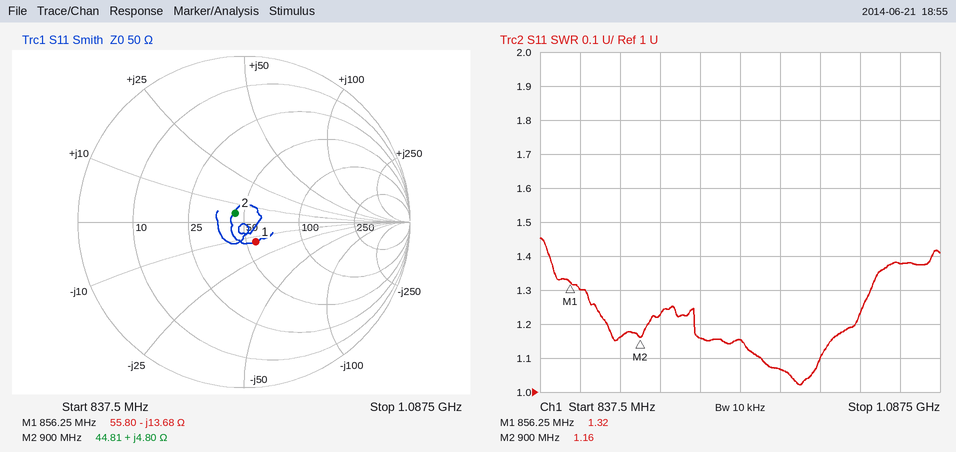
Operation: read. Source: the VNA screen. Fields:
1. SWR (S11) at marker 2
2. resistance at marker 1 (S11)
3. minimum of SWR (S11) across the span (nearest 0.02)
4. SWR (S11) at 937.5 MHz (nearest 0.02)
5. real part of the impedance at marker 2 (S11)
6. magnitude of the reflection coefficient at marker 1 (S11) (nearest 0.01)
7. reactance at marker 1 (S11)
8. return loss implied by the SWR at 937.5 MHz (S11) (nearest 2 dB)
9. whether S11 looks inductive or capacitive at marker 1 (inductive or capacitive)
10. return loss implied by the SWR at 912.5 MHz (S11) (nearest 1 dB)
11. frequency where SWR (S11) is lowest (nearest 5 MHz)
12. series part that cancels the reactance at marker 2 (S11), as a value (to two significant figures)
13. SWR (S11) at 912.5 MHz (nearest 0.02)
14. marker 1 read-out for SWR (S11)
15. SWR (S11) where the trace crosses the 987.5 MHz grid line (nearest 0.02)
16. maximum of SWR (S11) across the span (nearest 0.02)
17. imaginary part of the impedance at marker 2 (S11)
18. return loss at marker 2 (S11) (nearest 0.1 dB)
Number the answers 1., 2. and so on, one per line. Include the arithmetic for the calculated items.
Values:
1. 1.16
2. 55.80 Ω
3. 1.02
4. 1.16
5. 44.81 Ω
6. 0.14
7. -13.68 Ω
8. −20 log10((1.16 − 1)/(1.16 + 1)) ≈ 22.6 dB, so 22 dB to the nearest 2 dB
9. capacitive
10. −20 log10((1.22 − 1)/(1.22 + 1)) ≈ 20 dB
11. 1.000 GHz
12. C = 1/(2π × 900 MHz × 4.8 Ω) ≈ 37 pF
13. 1.22
14. 1.32
15. 1.06
16. 1.46
17. +4.80 Ω
18. 22.6 dB
